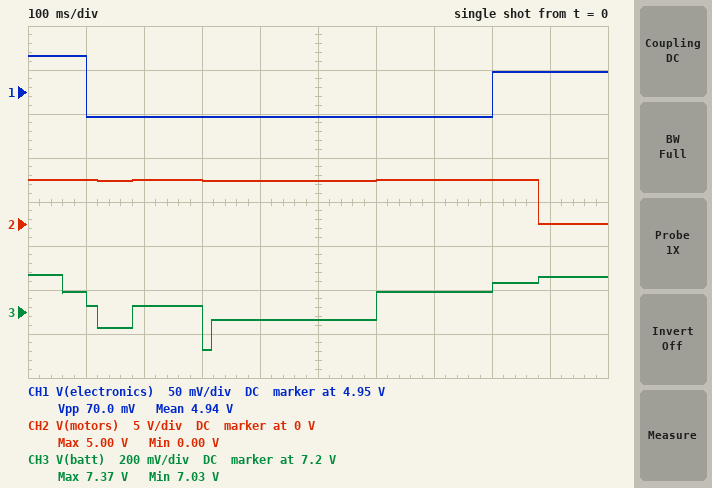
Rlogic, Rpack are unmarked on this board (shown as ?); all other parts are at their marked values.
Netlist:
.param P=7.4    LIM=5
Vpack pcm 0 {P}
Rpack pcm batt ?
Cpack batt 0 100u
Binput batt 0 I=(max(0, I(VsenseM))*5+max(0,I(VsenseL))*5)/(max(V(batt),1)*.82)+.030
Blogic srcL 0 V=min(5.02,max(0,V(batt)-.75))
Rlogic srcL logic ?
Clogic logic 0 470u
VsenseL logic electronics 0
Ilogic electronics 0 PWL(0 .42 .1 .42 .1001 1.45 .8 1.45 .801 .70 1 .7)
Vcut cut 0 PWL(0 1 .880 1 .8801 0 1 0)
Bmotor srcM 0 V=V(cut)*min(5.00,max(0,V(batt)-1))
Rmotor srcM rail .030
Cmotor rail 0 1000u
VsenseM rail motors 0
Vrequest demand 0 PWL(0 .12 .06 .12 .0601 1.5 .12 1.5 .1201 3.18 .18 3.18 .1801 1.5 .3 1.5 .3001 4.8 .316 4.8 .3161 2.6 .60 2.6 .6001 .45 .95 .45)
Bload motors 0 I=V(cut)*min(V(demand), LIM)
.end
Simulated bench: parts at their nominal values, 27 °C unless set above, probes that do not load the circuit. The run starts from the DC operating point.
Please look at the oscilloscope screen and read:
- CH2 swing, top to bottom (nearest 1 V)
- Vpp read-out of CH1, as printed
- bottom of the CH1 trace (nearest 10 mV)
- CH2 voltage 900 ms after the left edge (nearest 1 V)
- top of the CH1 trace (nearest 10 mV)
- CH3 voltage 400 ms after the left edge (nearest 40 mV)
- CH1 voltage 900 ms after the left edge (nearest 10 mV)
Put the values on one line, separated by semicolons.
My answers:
5 V; 70.0 mV; 4.92 V; 0 V; 4.99 V; 7.16 V; 4.97 V
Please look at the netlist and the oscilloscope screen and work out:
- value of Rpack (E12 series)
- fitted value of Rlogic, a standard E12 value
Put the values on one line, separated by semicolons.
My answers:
0.068 Ω; 0.068 Ω
